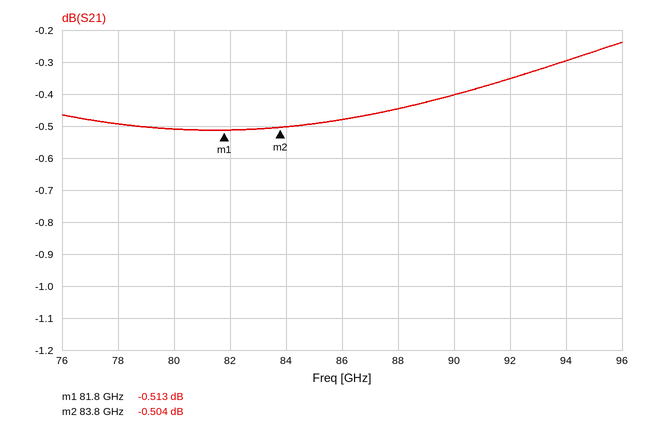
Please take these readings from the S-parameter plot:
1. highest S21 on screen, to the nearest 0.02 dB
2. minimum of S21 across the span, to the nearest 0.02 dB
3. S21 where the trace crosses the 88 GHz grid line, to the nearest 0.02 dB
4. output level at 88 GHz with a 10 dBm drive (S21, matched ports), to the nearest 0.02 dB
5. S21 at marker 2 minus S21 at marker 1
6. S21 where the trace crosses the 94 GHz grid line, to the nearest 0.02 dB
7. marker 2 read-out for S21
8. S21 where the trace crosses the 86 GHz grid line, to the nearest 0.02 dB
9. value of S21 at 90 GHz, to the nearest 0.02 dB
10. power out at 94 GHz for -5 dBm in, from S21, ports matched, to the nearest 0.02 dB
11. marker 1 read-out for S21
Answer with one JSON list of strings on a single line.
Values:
["-0.24 dB", "-0.52 dB", "-0.44 dB", "9.56 dBm", "0.009 dB", "-0.30 dB", "-0.504 dB", "-0.48 dB", "-0.40 dB", "-5.30 dBm", "-0.513 dB"]
